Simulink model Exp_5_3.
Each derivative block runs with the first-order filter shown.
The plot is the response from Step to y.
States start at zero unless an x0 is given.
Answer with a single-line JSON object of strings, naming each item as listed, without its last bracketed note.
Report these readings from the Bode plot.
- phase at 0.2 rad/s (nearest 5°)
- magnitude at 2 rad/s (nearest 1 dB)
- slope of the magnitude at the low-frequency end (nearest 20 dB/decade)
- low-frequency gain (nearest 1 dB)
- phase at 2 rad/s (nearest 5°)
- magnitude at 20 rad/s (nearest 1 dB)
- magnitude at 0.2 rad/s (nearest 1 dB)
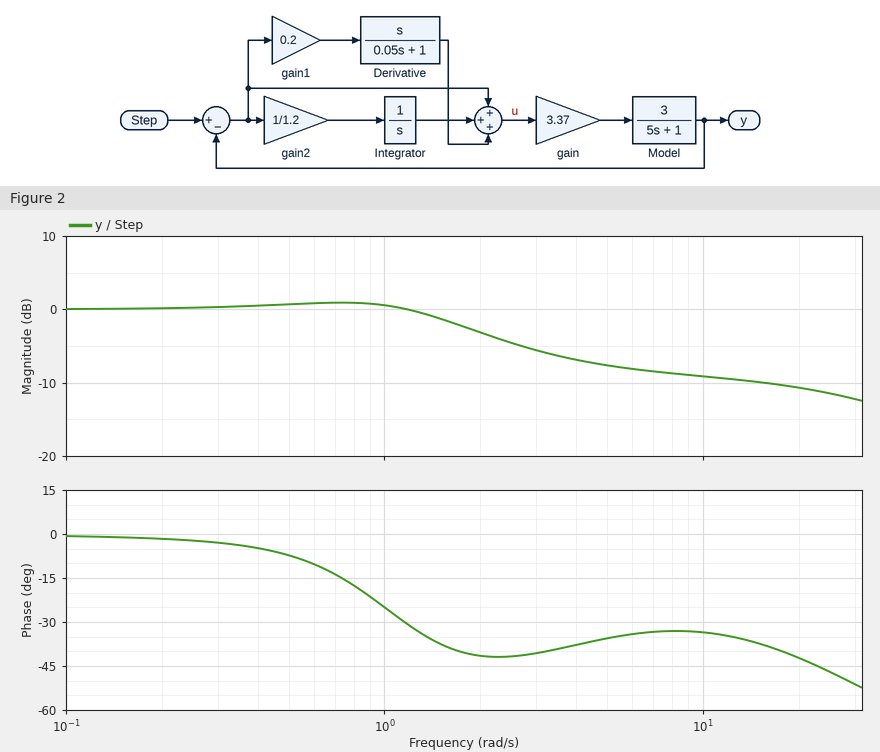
{"phase at 0.2 rad/s": "0°", "magnitude at 2 rad/s": "-3 dB", "slope of the magnitude at the low-frequency end": "0 dB/decade", "low-frequency gain": "0 dB", "phase at 2 rad/s": "-40°", "magnitude at 20 rad/s": "-11 dB", "magnitude at 0.2 rad/s": "0 dB"}
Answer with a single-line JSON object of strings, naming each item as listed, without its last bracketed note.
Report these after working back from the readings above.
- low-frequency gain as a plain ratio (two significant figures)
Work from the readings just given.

{"low-frequency gain as a plain ratio": "1.0"}
